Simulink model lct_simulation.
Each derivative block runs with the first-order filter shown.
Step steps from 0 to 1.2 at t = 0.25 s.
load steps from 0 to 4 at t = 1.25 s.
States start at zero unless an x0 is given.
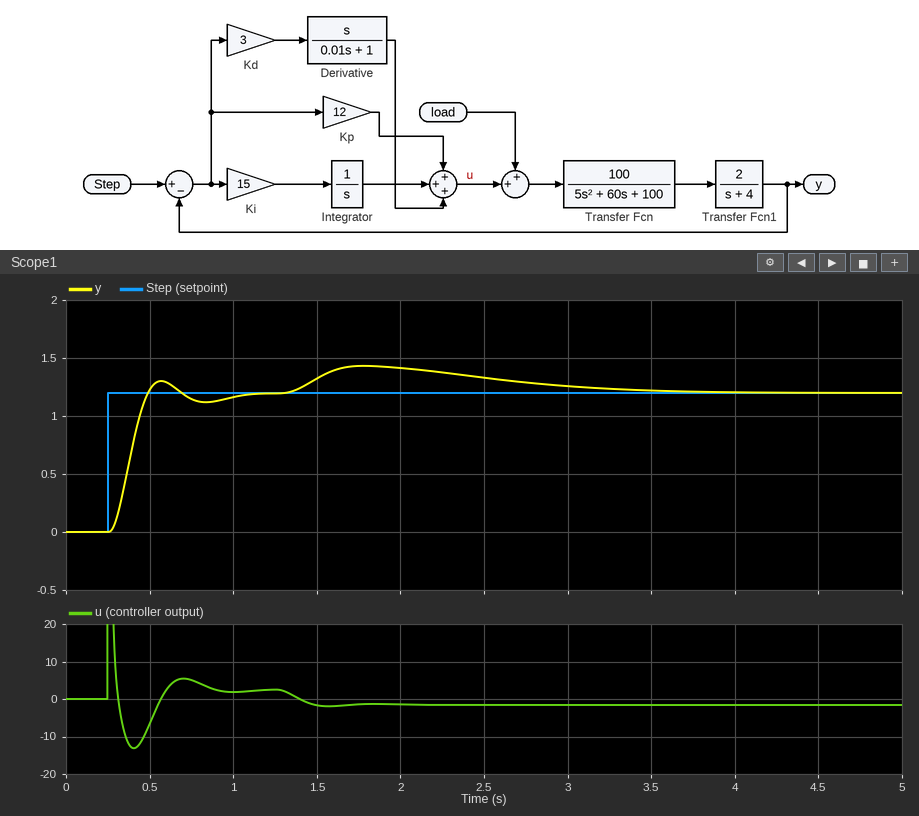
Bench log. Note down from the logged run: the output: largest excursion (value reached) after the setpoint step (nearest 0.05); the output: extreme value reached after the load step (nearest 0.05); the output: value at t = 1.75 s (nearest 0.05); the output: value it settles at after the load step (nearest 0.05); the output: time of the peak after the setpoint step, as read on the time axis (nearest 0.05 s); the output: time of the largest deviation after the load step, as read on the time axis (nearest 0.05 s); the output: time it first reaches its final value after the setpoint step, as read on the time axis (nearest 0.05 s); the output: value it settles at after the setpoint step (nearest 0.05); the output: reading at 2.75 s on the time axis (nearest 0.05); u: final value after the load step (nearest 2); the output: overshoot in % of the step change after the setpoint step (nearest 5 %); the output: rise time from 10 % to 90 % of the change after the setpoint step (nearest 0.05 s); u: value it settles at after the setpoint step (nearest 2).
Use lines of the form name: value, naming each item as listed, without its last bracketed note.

the output: largest excursion (value reached) after the setpoint step: 1.30
the output: extreme value reached after the load step: 1.45
the output: value at t = 1.75 s: 1.45
the output: value it settles at after the load step: 1.20
the output: time of the peak after the setpoint step, as read on the time axis: 0.55 s
the output: time of the largest deviation after the load step, as read on the time axis: 1.80 s
the output: time it first reaches its final value after the setpoint step, as read on the time axis: 0.50 s
the output: value it settles at after the setpoint step: 1.20
the output: reading at 2.75 s on the time axis: 1.30
u: final value after the load step: -2
the output: overshoot in % of the step change after the setpoint step: 10 %
the output: rise time from 10 % to 90 % of the change after the setpoint step: 0.15 s
u: value it settles at after the setpoint step: 2
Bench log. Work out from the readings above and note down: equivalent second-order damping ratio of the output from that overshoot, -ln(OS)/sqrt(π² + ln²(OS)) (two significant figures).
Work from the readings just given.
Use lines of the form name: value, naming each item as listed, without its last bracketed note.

equivalent second-order damping ratio of the output from that overshoot, -ln(OS)/sqrt(π² + ln²(OS)): 0.59
